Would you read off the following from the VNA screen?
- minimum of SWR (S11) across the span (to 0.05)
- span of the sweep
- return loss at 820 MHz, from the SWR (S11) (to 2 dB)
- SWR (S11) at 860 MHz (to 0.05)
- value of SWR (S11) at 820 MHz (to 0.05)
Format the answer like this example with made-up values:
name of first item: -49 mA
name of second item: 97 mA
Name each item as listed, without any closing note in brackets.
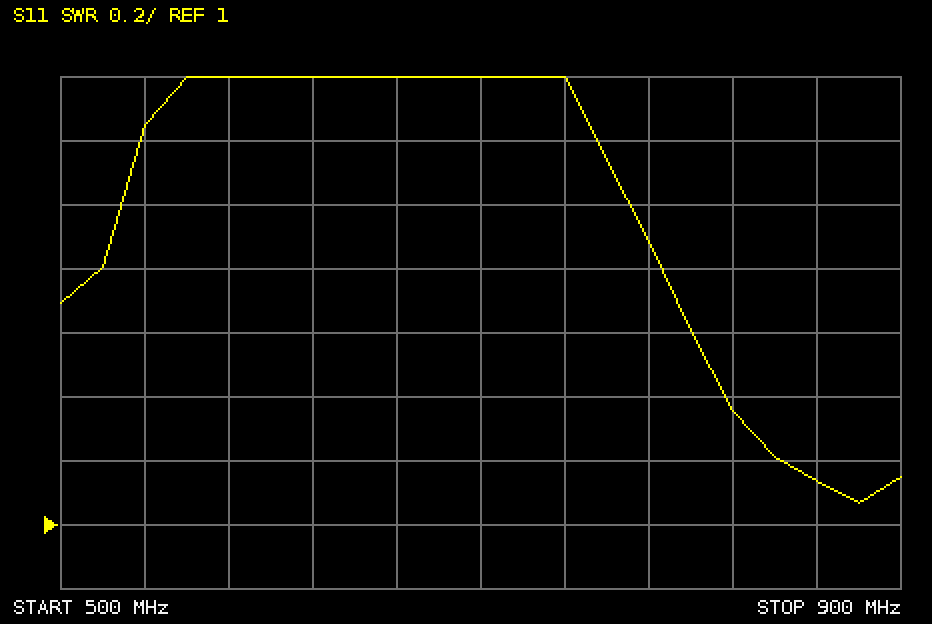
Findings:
minimum of SWR (S11) across the span: 1.05
span of the sweep: 400 MHz
return loss at 820 MHz, from the SWR (S11): 16 dB
SWR (S11) at 860 MHz: 1.15
value of SWR (S11) at 820 MHz: 1.35
